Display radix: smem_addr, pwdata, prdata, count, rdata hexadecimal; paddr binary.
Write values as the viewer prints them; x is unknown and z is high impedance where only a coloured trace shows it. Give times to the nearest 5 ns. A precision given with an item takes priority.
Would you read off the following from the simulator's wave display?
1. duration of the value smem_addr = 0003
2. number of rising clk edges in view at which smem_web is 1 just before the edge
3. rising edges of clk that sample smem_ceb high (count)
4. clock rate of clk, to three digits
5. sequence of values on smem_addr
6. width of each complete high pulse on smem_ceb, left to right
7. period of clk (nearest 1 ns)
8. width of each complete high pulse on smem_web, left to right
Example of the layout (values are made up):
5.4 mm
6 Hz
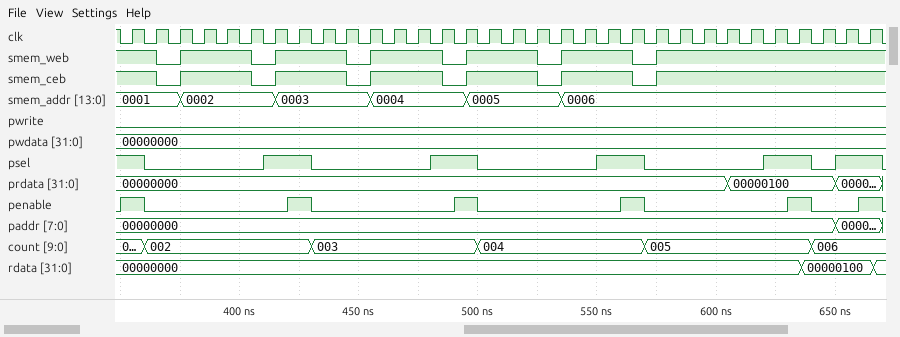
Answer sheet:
40 ns
26
26
100 MHz
0001, 0002, 0003, 0004, 0005, 0006
30 ns, 30 ns, 30 ns, 30 ns, 30 ns
10 ns
30 ns, 30 ns, 30 ns, 30 ns, 30 ns
